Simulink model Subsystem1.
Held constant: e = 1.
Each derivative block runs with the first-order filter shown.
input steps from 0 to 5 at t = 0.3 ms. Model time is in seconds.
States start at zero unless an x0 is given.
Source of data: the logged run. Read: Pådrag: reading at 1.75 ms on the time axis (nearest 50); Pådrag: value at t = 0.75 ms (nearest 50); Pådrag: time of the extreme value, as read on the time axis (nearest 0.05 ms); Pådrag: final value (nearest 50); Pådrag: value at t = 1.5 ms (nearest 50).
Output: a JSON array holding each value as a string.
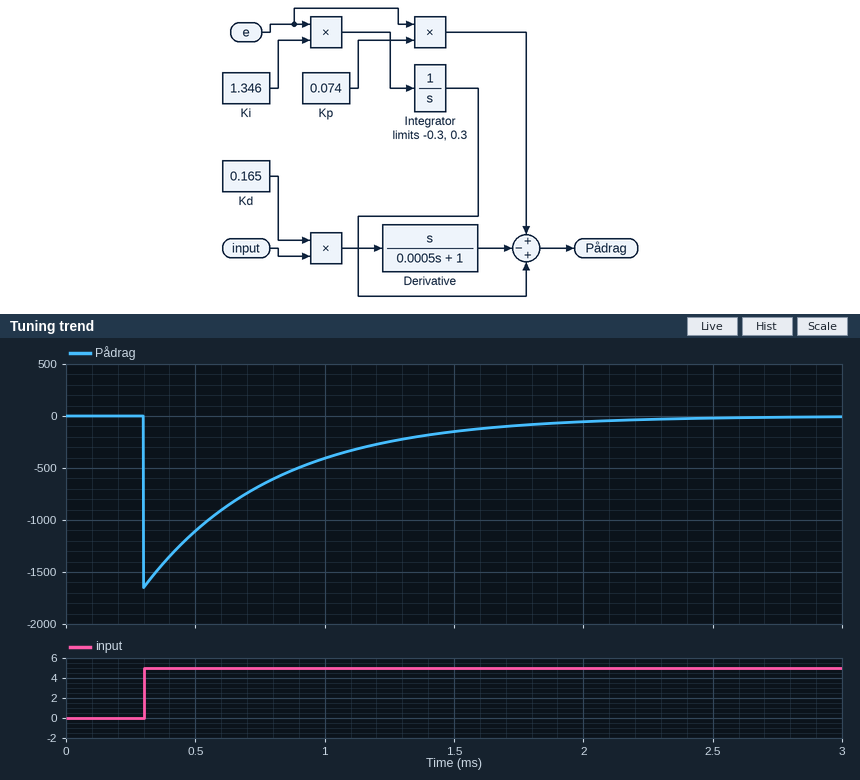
["-100", "-650", "0.30 ms", "0", "-150"]
